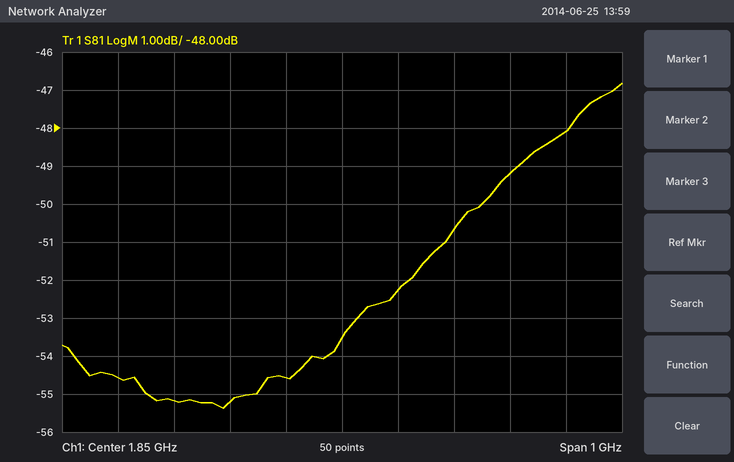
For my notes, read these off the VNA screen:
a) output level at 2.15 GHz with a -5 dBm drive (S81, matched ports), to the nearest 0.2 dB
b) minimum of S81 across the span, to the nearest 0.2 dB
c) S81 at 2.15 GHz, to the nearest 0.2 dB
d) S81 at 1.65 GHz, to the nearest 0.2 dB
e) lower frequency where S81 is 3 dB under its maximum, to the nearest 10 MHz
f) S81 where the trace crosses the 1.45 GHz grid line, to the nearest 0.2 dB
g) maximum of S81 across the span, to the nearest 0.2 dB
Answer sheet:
-54.2 dBm
-55.4 dB
-49.2 dB
-55.2 dB
2.11 GHz
-54.6 dB
-46.8 dB
